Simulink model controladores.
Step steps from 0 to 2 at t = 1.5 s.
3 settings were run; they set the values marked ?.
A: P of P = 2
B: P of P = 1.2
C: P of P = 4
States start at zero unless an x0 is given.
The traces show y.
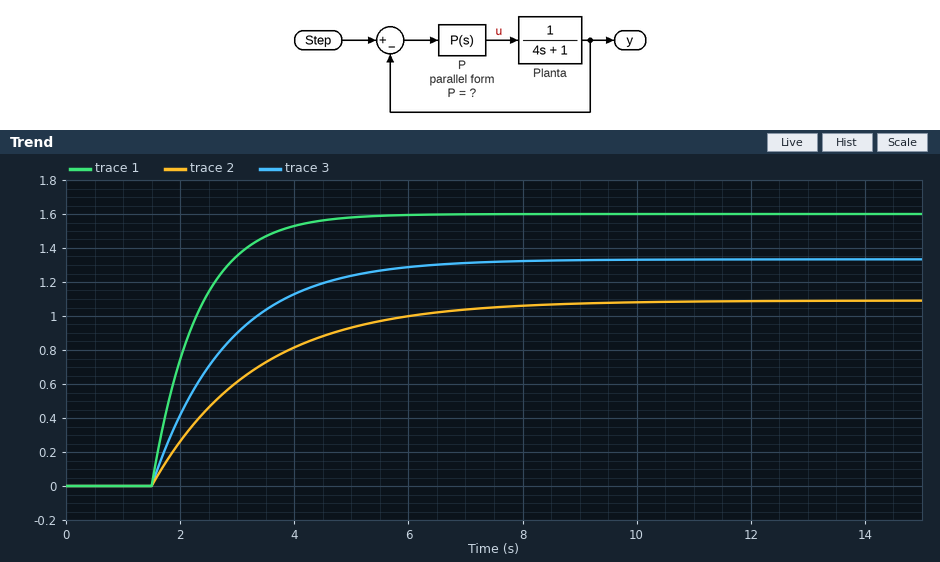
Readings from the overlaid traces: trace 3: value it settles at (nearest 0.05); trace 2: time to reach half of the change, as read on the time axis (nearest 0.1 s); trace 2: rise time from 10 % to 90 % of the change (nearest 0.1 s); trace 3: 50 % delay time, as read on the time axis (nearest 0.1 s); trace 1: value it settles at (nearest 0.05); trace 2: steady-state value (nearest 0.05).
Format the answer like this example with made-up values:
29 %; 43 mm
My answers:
1.35; 2.8 s; 4.0 s; 2.4 s; 1.60; 1.10
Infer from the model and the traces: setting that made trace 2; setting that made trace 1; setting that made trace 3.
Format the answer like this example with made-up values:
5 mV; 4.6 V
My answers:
B; C; A
